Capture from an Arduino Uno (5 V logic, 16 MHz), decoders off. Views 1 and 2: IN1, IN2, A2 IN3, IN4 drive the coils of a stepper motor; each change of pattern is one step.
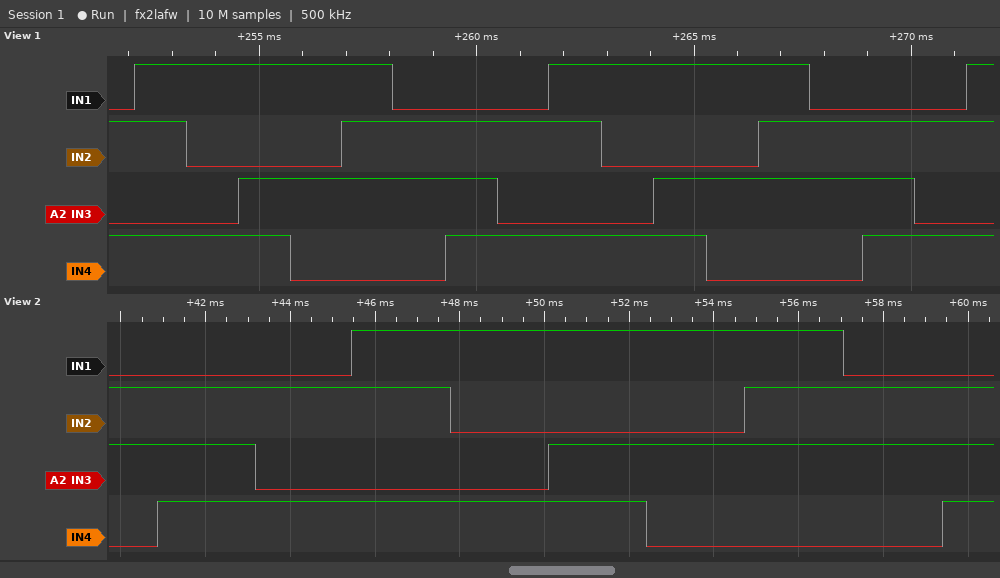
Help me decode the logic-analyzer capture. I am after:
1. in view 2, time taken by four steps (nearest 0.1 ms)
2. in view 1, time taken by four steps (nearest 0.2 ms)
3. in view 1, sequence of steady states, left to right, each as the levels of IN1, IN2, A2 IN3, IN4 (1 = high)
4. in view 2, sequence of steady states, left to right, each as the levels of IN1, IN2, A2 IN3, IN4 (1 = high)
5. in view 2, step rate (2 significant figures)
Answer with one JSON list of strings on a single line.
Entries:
["9.2 ms", "4.8 ms", "0101 1101 1001 1011 1010 1110 0110 0111 0101 1101 1001 1011 1010 1110 0110 0111 0101 1101", "0110 0111 0101 1101 1001 1011 1010 1110 0110 0111", "430 steps/s"]
